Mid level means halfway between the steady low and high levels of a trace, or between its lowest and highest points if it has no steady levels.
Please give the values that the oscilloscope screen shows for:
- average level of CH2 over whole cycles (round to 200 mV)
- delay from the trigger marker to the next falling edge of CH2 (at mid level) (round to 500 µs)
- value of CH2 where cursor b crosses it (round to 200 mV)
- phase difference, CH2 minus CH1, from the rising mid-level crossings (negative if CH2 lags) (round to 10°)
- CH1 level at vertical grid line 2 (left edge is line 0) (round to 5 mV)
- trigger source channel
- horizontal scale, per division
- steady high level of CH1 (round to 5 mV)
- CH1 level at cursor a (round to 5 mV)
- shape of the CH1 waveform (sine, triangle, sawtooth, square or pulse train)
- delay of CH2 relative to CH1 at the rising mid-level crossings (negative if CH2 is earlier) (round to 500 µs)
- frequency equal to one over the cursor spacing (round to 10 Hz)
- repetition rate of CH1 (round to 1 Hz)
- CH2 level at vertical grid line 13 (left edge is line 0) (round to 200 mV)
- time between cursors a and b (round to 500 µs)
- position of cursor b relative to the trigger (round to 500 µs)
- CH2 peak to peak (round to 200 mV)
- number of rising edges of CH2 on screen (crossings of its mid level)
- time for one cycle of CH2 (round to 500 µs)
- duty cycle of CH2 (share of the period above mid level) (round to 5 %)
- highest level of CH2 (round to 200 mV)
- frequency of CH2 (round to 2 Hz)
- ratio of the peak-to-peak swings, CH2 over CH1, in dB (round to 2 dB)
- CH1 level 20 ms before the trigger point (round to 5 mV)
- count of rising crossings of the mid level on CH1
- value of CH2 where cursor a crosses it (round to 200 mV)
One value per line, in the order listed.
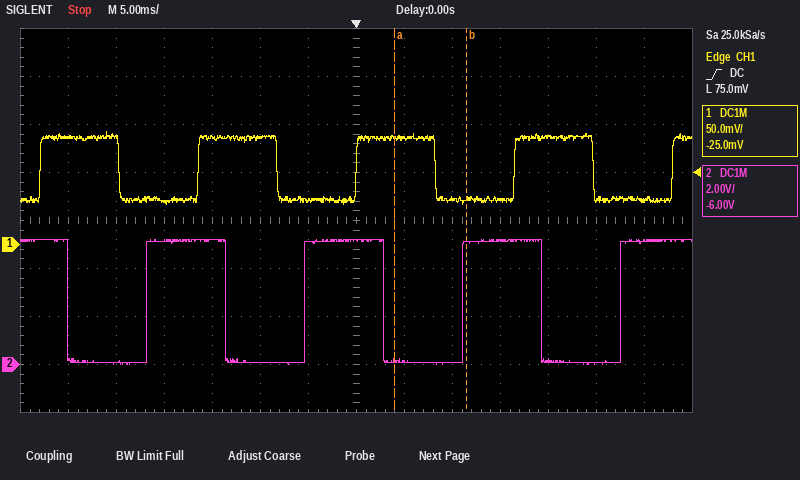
2.6 V
3.0 ms
5.0 V
+120°
110 mV
CH1
5 ms
110 mV
110 mV
square
-5.5 ms
130 Hz
61 Hz
5.2 V
7.5 ms
+11.5 ms
5.2 V
4
16.5 ms
50 %
5.2 V
60 Hz
36 dB
45 mV
5
200 mV
